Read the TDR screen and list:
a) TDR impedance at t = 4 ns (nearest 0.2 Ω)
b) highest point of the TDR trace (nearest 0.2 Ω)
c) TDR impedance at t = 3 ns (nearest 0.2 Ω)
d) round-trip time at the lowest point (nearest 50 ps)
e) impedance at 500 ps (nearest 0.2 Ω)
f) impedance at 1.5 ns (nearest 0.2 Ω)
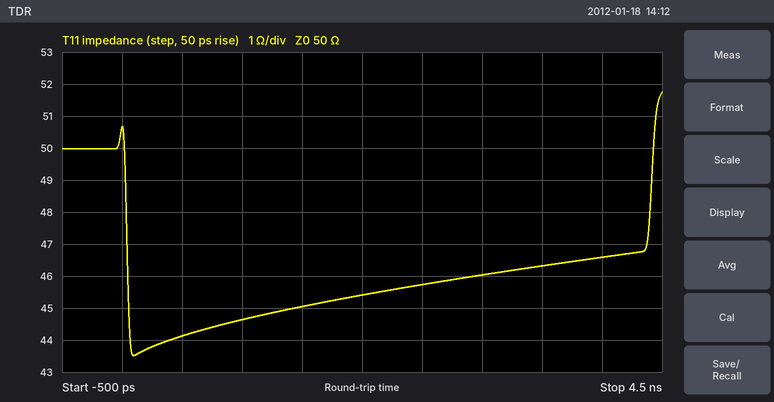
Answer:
46.6 Ω
51.8 Ω
46.0 Ω
100 ps
44.2 Ω
45.0 Ω
